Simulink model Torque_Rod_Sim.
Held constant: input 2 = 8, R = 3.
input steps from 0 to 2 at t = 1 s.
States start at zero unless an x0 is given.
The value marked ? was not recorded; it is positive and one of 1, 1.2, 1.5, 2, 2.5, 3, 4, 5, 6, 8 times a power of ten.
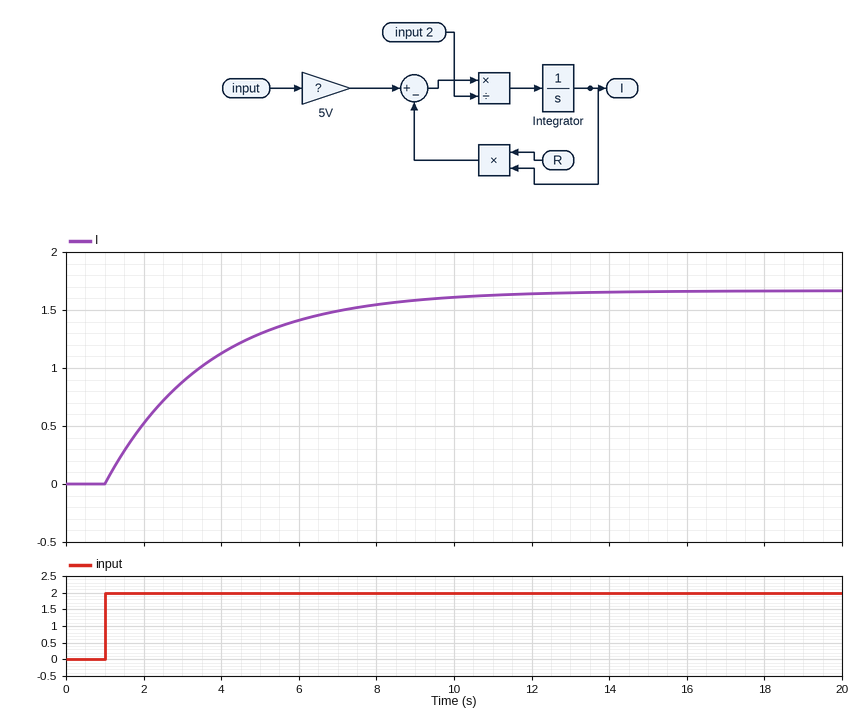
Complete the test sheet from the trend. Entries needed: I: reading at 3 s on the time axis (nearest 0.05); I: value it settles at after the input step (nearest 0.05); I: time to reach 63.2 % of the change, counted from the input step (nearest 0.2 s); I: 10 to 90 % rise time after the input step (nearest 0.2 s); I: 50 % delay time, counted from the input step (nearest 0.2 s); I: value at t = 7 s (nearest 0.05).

0.90
1.65
2.6 s
5.8 s
1.8 s
1.50
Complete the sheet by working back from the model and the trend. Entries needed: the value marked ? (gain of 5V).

2.5
